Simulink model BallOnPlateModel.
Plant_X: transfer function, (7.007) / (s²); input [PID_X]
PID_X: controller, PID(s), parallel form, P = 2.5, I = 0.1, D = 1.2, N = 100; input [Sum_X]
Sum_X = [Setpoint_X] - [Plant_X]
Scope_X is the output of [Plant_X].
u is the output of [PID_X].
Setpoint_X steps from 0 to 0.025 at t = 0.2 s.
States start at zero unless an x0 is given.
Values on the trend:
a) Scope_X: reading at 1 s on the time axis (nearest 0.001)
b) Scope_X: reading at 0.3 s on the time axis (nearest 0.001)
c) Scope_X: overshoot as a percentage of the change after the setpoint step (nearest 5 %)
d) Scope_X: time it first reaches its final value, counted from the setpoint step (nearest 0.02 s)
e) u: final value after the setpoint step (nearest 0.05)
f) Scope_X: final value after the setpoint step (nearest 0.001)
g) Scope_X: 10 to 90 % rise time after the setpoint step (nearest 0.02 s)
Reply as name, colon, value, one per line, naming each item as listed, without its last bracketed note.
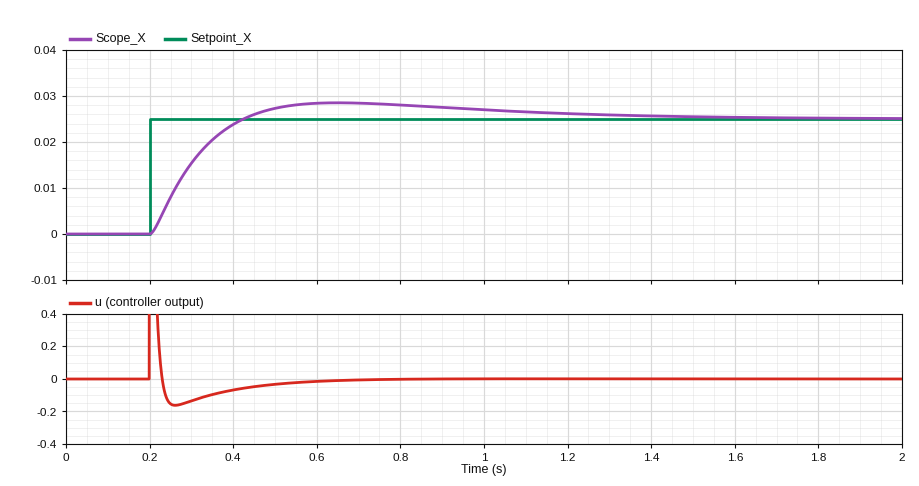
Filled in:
Scope_X: reading at 1 s on the time axis: 0.027
Scope_X: reading at 0.3 s on the time axis: 0.015
Scope_X: overshoot as a percentage of the change after the setpoint step: 15 %
Scope_X: time it first reaches its final value, counted from the setpoint step: 0.22 s
u: final value after the setpoint step: 0.00
Scope_X: final value after the setpoint step: 0.025
Scope_X: 10 to 90 % rise time after the setpoint step: 0.16 s
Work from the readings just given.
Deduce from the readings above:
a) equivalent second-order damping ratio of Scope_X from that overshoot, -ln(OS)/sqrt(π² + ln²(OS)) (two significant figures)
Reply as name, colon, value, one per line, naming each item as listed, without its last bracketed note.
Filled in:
equivalent second-order damping ratio of Scope_X from that overshoot, -ln(OS)/sqrt(π² + ln²(OS)): 0.52
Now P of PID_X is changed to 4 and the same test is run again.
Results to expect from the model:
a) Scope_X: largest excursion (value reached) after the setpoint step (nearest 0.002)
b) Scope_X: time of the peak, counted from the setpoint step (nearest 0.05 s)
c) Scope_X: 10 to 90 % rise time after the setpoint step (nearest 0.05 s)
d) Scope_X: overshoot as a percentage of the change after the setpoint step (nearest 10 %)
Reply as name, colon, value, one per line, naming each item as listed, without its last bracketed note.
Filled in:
Scope_X: largest excursion (value reached) after the setpoint step: 0.030
Scope_X: time of the peak, counted from the setpoint step: 0.40 s
Scope_X: 10 to 90 % rise time after the setpoint step: 0.15 s
Scope_X: overshoot as a percentage of the change after the setpoint step: 20 %
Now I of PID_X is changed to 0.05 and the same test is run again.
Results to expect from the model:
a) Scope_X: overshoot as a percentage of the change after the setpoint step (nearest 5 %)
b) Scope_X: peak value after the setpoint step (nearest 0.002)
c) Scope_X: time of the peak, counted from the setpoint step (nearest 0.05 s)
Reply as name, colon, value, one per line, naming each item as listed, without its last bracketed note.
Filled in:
Scope_X: overshoot as a percentage of the change after the setpoint step: 15 %
Scope_X: peak value after the setpoint step: 0.028
Scope_X: time of the peak, counted from the setpoint step: 0.45 s
